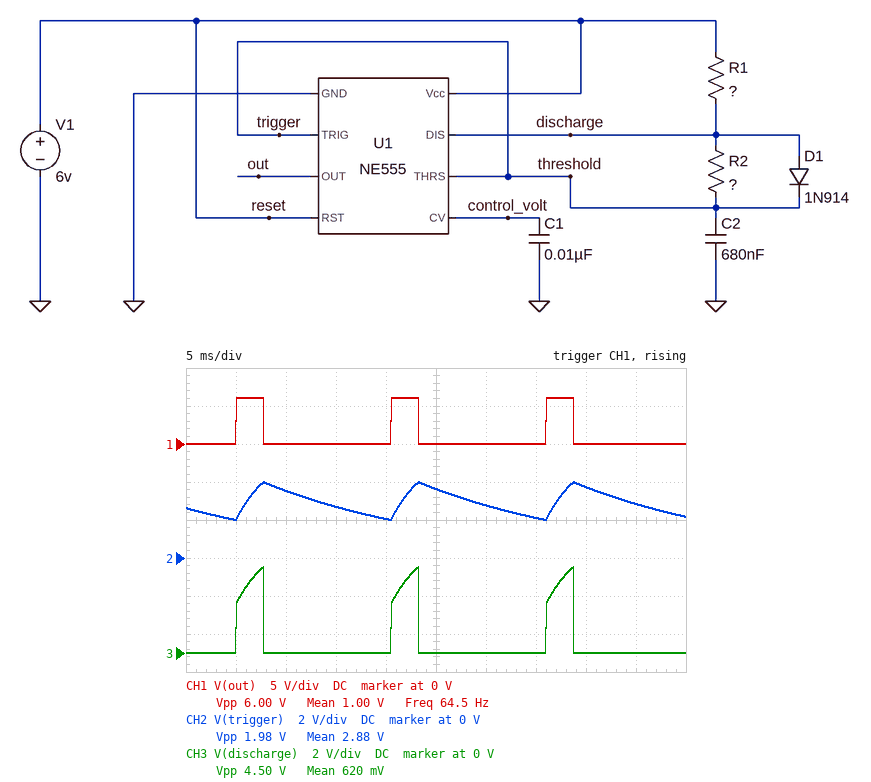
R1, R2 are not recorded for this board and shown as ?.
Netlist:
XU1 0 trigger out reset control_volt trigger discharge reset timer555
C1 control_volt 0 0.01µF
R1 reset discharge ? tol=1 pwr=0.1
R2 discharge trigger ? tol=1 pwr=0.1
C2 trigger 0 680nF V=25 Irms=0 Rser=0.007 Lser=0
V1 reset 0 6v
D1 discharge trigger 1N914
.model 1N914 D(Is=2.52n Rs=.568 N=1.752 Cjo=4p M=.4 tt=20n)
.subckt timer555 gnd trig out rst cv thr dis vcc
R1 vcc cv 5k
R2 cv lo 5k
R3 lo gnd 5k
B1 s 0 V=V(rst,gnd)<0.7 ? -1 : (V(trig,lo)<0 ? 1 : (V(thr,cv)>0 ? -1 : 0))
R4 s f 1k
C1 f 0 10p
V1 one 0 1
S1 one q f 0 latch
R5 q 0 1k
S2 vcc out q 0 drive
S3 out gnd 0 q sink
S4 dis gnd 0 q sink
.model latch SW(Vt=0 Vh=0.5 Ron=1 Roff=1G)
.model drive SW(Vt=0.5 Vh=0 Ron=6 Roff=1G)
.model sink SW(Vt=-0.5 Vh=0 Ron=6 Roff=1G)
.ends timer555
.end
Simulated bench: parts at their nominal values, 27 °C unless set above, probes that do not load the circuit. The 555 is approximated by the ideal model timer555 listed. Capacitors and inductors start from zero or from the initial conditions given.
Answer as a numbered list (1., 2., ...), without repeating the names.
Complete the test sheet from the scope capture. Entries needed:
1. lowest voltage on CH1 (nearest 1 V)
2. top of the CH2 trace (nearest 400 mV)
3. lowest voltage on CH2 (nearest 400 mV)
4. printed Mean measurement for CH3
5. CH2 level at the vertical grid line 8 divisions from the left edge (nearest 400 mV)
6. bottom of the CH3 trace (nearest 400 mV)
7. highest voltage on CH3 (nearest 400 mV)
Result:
1. 0 V
2. 4.0 V
3. 2.0 V
4. 620 mV
5. 3.6 V
6. 0 V
7. 4.4 V
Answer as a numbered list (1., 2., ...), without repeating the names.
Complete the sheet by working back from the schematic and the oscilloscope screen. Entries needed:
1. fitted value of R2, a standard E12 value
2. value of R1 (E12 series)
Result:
1. 27 kΩ
2. 4.7 kΩ
